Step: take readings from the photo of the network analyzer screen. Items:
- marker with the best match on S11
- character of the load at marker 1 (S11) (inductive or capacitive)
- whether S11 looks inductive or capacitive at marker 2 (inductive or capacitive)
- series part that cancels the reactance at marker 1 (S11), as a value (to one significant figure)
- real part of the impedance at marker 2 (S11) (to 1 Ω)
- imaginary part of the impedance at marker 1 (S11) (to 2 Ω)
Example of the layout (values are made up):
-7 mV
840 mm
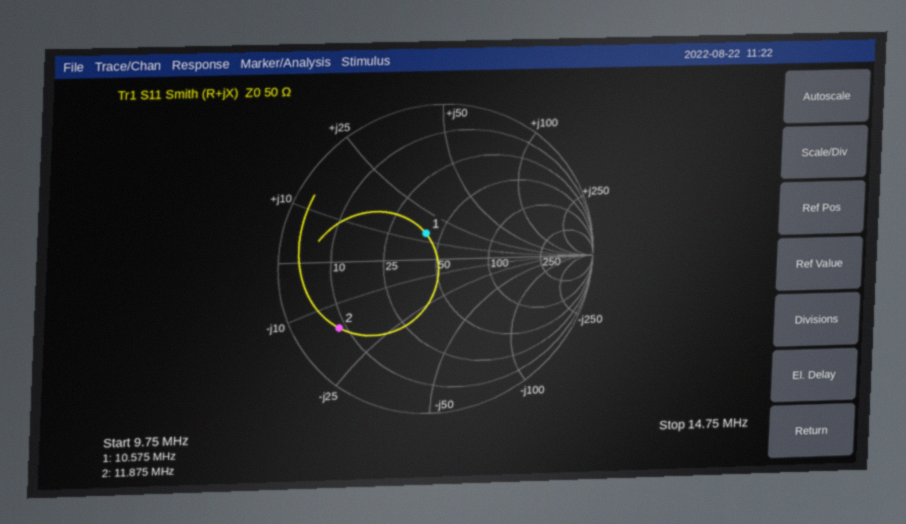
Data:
marker 1
inductive
capacitive
1 nF
8 Ω
+14 Ω
